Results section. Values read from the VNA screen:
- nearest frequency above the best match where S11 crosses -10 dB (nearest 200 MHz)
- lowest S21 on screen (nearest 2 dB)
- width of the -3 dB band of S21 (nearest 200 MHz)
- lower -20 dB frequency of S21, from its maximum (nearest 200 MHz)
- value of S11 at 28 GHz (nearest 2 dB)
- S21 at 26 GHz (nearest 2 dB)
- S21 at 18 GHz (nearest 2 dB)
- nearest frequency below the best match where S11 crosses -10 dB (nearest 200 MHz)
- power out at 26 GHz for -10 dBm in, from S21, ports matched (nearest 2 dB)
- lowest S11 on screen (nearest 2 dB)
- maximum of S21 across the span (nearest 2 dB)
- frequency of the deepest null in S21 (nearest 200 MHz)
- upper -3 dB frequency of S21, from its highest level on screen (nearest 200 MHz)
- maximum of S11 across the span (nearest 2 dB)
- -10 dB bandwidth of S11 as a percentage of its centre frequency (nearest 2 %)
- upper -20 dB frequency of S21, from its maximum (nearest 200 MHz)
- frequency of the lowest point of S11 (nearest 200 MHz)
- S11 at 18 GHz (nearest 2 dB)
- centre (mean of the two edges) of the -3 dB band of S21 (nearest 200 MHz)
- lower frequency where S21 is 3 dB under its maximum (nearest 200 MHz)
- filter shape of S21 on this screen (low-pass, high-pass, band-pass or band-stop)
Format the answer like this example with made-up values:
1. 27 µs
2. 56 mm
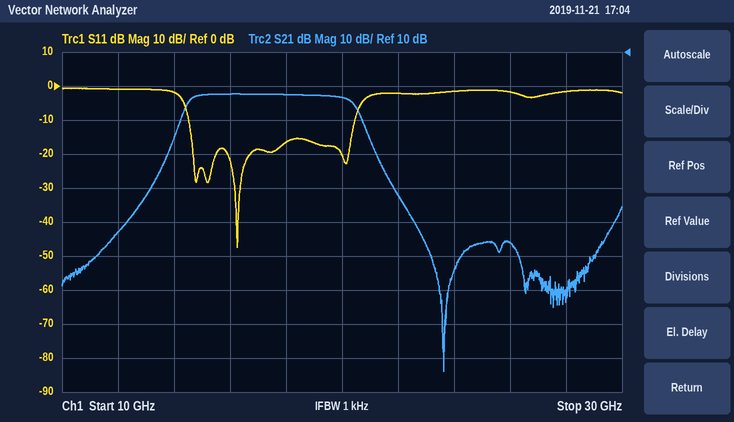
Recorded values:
1. 20.4 GHz
2. -84 dB
3. 6.0 GHz
4. 13.6 GHz
5. -2 dB
6. -46 dB
7. -2 dB
8. 14.6 GHz
9. -56 dBm
10. -48 dB
11. -2 dB
12. 23.6 GHz
13. 20.4 GHz
14. 0 dB
15. 34 %
16. 21.4 GHz
17. 16.2 GHz
18. -16 dB
19. 17.4 GHz
20. 14.4 GHz
21. band-pass
